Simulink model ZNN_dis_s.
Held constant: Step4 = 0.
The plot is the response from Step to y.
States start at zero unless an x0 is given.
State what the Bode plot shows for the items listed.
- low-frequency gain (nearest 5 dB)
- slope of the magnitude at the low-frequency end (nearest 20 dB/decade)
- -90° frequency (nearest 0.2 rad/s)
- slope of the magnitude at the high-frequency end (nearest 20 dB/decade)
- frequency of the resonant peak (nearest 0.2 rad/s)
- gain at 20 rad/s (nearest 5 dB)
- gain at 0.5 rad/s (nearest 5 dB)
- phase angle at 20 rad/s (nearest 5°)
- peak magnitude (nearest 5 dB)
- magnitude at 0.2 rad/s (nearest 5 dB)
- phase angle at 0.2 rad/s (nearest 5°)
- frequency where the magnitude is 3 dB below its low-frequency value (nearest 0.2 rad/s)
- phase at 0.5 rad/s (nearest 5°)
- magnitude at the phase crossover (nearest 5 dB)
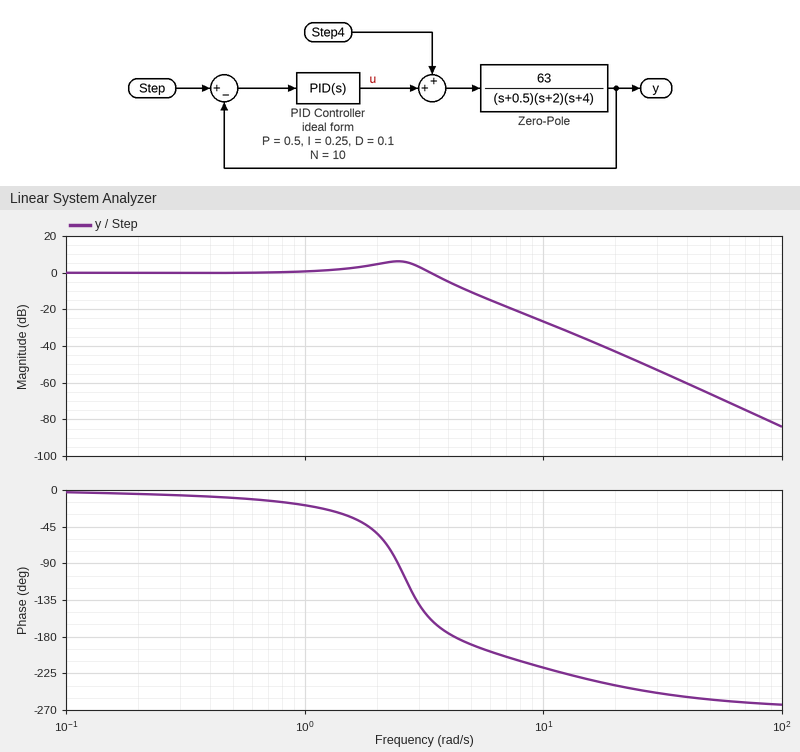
0 dB
0 dB/decade
2.4 rad/s
-60 dB/decade
2.4 rad/s
-45 dB
0 dB
-240°
5 dB
0 dB
-5°
3.8 rad/s
-10°
-5 dB
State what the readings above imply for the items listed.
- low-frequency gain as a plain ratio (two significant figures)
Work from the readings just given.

1.0
